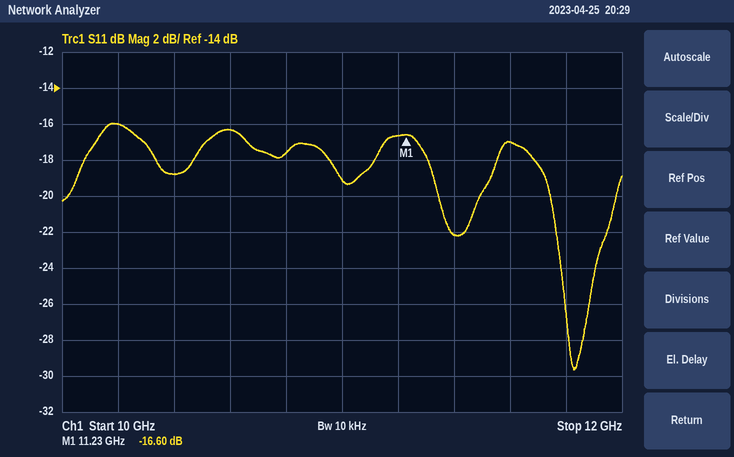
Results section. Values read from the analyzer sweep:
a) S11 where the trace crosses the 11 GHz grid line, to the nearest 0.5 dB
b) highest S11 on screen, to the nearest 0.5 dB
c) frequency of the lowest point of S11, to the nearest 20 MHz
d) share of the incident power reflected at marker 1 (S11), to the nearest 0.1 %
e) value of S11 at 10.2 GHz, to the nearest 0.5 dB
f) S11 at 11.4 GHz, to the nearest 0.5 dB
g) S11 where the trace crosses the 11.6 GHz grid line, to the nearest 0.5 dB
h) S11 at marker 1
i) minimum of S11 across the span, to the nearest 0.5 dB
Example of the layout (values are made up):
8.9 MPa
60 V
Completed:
-19.0 dB
-16.0 dB
11.82 GHz
2.2 %
-16.0 dB
-22.0 dB
-17.0 dB
-16.60 dB
-29.5 dB
